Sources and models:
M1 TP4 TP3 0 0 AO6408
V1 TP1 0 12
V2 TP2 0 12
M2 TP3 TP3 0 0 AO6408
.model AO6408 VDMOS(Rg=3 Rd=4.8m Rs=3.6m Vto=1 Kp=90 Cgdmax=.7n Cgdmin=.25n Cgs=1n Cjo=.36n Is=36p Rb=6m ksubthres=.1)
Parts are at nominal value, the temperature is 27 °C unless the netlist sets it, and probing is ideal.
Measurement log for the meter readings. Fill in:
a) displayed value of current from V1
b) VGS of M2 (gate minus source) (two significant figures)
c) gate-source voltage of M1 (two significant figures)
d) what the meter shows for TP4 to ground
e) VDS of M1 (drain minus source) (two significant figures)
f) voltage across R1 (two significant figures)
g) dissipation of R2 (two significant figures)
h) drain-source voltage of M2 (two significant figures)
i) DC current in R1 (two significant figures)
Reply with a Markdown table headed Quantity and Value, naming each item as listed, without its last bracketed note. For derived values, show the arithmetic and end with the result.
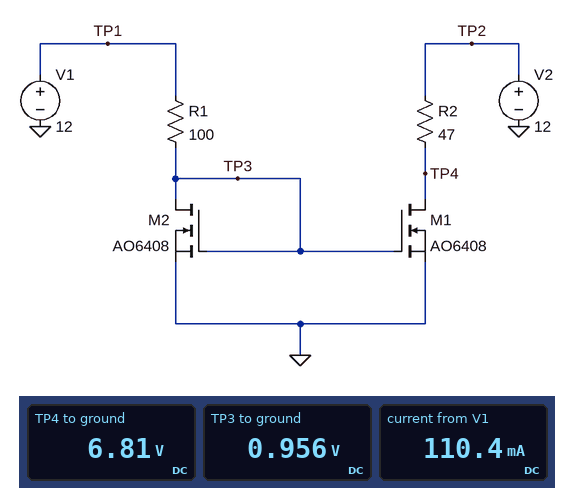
| Quantity | Value |
|---|---|
| displayed value of current from V1 | 110.4 mA |
| VGS of M2 (gate minus source) | 956 mV = 960 mV |
| gate-source voltage of M1 | 956 mV = 960 mV |
| what the meter shows for TP4 to ground | 6.81 V |
| VDS of M1 (drain minus source) | 6.81 V = 6.8 V |
| voltage across R1 | 12 V - 956 mV = 11 V |
| dissipation of R2 | (12 V - 6.81 V)^2 / 47 Ω = 570 mW |
| drain-source voltage of M2 | 956 mV = 960 mV |
| DC current in R1 | (12 V - 956 mV) / 100 Ω = 110 mA |
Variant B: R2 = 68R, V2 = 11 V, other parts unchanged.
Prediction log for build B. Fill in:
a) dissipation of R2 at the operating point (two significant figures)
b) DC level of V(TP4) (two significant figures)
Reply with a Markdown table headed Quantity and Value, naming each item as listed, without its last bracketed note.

| Quantity | Value |
|---|---|
| dissipation of R2 at the operating point | 830 mW |
| DC level of V(TP4) | 3.5 V |
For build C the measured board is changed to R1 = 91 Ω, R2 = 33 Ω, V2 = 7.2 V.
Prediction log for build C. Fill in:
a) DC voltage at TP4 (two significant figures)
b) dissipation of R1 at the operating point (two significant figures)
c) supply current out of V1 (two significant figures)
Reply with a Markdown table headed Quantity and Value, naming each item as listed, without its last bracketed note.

| Quantity | Value |
|---|---|
| DC voltage at TP4 | 3.2 V |
| dissipation of R1 at the operating point | 1.3 W |
| supply current out of V1 | 120 mA |
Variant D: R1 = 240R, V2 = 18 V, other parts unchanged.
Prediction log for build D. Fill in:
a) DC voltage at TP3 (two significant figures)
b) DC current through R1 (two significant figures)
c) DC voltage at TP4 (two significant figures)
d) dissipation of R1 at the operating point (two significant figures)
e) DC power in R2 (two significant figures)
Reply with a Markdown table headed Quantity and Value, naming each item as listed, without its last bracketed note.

| Quantity | Value |
|---|---|
| DC voltage at TP3 | 900 mV |
| DC current through R1 | 46 mA |
| DC voltage at TP4 | 16 V |
| dissipation of R1 at the operating point | 510 mW |
| DC power in R2 | 100 mW |
